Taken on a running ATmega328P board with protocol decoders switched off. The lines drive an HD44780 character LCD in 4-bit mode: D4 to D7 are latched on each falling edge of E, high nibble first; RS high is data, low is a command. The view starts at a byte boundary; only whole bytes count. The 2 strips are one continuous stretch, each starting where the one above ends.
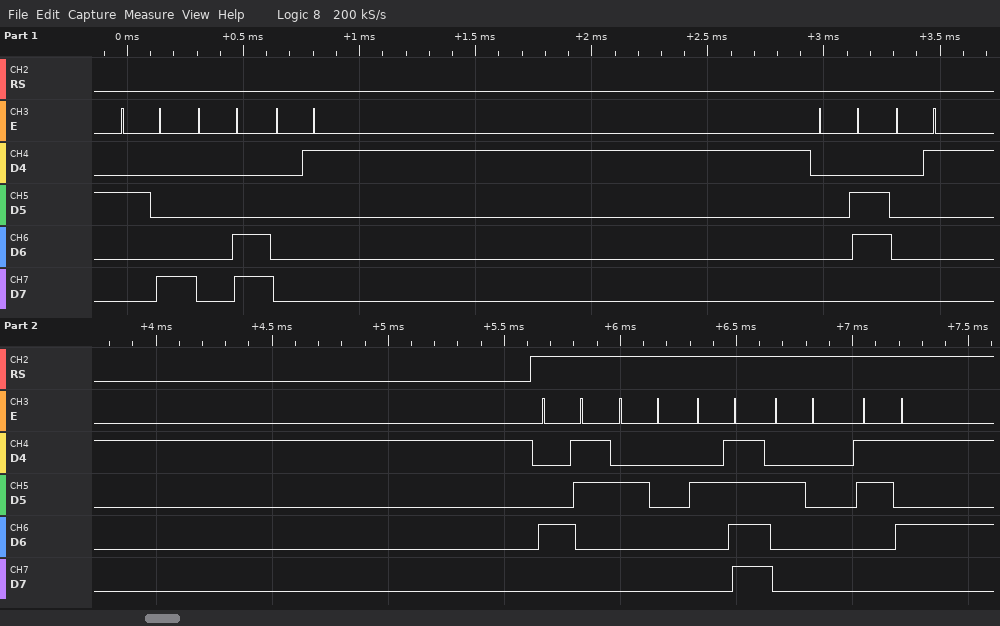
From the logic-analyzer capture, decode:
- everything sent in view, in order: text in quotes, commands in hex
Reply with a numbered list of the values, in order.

1. 0x28 0x0C 0x01 0x06 0x01 "C / 5"
